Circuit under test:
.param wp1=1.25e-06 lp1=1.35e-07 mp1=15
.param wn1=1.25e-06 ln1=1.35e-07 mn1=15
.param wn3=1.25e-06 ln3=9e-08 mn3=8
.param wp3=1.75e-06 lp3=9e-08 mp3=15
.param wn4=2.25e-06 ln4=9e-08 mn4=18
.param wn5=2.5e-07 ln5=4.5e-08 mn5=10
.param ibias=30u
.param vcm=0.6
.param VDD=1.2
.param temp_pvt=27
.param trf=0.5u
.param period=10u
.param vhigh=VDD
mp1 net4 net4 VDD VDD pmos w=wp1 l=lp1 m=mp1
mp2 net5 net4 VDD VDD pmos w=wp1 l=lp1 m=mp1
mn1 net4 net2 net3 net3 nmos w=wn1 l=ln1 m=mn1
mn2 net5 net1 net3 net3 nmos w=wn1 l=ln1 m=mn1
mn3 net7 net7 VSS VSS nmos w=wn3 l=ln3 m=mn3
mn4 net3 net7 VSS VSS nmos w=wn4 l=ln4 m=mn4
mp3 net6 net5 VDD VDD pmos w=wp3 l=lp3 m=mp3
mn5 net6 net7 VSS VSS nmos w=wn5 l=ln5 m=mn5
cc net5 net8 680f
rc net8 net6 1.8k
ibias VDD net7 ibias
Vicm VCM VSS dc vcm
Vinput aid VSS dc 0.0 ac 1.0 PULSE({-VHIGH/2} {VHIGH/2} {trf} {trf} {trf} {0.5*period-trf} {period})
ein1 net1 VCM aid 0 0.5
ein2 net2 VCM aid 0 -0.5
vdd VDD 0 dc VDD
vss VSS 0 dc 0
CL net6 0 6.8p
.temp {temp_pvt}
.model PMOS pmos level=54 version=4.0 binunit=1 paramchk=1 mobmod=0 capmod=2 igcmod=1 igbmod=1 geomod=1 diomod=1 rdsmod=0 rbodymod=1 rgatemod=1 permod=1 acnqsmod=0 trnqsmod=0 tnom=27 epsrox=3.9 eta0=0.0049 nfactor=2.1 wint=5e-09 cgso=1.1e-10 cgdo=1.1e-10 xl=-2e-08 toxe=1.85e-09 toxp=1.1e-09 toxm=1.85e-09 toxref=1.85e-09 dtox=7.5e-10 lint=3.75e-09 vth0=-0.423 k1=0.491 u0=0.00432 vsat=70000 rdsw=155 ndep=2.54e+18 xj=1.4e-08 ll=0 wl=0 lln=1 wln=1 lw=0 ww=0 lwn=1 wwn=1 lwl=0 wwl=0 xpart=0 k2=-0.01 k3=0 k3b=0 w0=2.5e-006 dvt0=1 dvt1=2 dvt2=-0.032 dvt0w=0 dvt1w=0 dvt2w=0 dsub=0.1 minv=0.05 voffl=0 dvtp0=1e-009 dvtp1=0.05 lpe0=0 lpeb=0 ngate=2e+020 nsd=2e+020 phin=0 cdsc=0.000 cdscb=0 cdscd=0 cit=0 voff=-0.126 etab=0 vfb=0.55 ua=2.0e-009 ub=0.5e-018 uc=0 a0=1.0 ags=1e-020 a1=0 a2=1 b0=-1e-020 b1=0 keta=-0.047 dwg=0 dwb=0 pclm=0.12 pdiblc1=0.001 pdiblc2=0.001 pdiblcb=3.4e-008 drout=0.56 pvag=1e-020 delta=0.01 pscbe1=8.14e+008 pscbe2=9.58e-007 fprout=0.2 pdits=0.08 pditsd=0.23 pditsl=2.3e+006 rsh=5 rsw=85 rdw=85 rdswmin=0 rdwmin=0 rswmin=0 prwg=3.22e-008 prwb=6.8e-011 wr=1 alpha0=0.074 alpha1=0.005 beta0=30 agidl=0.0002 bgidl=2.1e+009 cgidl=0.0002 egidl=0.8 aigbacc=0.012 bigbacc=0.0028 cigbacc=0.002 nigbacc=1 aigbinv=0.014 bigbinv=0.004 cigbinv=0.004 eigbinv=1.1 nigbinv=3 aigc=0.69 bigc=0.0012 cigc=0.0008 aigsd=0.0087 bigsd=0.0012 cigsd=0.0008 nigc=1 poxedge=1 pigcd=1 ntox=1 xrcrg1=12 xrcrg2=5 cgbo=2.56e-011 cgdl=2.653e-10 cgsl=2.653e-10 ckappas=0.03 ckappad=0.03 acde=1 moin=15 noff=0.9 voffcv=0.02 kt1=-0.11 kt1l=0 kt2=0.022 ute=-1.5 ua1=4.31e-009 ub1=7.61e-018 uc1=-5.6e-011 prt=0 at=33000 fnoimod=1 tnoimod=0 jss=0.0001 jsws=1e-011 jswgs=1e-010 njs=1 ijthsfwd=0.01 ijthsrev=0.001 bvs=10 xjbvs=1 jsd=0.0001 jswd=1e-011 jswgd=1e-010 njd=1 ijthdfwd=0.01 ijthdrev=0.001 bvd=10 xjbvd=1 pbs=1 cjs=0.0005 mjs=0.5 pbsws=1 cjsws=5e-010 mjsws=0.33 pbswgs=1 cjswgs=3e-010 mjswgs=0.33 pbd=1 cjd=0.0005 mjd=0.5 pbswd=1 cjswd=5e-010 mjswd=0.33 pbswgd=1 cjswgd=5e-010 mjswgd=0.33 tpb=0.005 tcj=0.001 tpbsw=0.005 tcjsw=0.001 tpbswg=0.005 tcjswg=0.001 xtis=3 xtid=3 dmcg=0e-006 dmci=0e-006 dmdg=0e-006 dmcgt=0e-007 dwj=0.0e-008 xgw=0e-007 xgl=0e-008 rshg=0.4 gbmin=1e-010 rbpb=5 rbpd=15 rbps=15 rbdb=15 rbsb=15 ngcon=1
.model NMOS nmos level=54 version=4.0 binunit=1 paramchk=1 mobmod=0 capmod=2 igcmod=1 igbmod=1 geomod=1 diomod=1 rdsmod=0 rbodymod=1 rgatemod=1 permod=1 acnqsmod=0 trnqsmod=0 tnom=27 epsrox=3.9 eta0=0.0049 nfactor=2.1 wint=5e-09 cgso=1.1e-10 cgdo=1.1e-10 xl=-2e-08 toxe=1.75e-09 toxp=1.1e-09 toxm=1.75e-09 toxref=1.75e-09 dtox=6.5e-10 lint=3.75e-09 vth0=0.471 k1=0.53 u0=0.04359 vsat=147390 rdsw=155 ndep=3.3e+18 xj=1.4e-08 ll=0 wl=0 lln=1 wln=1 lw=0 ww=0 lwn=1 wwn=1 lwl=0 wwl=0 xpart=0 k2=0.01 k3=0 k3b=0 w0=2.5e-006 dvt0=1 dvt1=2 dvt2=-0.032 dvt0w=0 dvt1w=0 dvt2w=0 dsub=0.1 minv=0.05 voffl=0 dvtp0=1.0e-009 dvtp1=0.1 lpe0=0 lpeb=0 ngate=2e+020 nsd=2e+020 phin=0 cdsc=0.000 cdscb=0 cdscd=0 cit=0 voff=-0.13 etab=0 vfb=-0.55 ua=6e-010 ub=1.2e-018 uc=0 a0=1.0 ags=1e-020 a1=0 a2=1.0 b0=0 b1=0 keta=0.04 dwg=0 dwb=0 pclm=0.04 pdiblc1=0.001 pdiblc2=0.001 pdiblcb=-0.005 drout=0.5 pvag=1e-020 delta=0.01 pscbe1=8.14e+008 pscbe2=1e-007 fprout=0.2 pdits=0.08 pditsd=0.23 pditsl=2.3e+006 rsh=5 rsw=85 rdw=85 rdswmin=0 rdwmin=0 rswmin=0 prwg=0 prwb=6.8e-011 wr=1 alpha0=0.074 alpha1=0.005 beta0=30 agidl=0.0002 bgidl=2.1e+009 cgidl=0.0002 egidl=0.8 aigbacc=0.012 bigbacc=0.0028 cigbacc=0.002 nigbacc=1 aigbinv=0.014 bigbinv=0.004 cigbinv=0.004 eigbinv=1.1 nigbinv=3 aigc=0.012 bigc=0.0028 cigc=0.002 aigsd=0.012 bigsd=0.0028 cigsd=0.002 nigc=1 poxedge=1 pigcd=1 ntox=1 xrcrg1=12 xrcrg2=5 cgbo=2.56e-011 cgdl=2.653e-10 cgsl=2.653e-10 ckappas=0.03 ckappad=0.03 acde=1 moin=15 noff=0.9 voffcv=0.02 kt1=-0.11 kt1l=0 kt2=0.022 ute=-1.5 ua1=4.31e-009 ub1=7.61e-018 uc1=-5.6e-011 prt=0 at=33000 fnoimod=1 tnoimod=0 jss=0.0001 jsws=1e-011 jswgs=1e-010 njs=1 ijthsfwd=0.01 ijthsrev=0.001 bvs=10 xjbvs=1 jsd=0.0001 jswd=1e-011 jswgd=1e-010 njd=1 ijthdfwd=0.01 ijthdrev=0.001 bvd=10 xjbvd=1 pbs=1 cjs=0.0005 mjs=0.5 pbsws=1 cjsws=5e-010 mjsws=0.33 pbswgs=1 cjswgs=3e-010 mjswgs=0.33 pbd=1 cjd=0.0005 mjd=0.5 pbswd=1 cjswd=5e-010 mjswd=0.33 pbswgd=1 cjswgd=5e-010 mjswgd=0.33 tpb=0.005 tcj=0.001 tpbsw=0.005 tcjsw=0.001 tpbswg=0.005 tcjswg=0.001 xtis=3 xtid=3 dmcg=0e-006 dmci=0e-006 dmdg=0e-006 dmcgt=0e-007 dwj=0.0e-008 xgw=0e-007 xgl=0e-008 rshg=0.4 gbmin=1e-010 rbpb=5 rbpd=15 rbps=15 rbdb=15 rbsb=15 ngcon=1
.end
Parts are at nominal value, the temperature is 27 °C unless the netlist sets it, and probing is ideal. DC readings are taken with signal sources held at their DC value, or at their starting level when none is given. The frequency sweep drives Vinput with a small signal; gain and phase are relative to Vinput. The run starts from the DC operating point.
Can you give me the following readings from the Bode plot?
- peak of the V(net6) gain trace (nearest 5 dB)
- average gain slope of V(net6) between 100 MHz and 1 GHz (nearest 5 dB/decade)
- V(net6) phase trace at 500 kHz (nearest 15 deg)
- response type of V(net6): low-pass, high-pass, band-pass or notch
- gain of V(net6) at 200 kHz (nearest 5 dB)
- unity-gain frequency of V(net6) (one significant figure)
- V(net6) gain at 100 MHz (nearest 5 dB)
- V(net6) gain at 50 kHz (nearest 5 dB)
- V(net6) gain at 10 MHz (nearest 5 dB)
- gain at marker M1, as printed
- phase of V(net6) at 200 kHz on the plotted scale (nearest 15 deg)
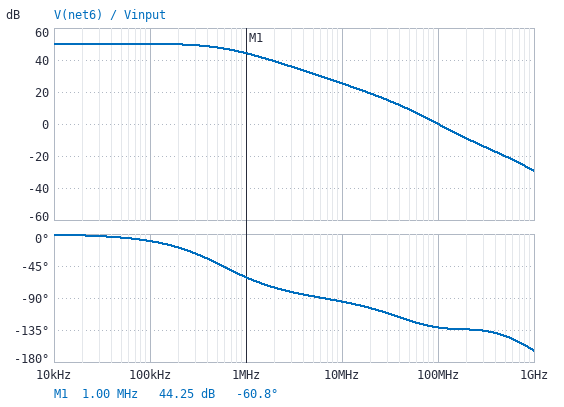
50 dB
-30 dB/decade
-45 deg
low-pass
50 dB
100 MHz
0 dB
50 dB
25 dB
44.25 dB
-15 deg
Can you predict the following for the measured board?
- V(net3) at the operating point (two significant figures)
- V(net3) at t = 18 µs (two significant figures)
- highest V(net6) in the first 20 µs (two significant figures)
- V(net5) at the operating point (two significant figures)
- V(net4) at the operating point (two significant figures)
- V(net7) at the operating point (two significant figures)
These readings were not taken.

180 mV
440 mV
1.2 V
680 mV
680 mV
390 mV
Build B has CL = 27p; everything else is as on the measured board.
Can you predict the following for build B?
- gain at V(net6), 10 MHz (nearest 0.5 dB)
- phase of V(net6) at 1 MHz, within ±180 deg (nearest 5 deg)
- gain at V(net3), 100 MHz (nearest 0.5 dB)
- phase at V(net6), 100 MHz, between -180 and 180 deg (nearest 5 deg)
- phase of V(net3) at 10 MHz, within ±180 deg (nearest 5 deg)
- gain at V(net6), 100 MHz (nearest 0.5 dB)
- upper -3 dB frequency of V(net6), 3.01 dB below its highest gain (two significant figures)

22.5 dB
-65 deg
-39.5 dB
-150 deg
140 deg
-11.0 dB
500 kHz
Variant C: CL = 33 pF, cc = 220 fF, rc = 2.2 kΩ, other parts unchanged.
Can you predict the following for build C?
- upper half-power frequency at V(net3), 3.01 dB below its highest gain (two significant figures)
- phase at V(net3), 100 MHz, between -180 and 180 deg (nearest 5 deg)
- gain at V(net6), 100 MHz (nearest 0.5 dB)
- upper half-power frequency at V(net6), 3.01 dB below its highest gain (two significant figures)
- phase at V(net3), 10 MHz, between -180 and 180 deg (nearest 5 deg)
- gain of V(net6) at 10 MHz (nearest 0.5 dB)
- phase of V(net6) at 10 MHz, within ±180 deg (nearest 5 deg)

1.4 MHz
130 deg
-6.0 dB
970 kHz
145 deg
28.5 dB
-115 deg
